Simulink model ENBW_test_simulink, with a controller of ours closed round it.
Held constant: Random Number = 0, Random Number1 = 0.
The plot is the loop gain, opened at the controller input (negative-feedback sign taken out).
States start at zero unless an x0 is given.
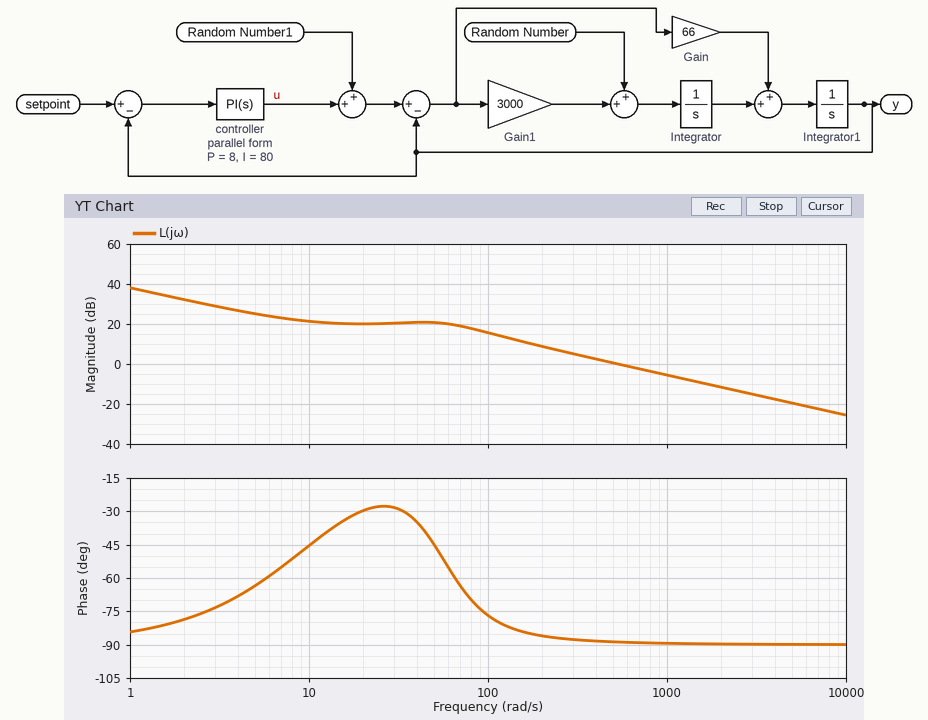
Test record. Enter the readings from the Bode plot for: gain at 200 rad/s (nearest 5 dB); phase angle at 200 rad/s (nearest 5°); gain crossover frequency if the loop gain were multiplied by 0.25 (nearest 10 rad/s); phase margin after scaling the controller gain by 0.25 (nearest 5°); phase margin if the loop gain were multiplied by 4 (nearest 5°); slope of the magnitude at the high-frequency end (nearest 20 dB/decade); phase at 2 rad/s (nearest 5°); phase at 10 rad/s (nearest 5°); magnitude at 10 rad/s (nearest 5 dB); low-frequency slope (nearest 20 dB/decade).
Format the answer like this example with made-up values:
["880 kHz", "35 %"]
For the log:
["10 dB", "-85°", "140 rad/s", "95°", "90°", "-20 dB/decade", "-80°", "-45°", "20 dB", "-20 dB/decade"]
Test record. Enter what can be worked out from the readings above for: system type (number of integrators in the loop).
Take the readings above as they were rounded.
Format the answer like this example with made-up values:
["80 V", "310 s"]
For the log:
["1"]
